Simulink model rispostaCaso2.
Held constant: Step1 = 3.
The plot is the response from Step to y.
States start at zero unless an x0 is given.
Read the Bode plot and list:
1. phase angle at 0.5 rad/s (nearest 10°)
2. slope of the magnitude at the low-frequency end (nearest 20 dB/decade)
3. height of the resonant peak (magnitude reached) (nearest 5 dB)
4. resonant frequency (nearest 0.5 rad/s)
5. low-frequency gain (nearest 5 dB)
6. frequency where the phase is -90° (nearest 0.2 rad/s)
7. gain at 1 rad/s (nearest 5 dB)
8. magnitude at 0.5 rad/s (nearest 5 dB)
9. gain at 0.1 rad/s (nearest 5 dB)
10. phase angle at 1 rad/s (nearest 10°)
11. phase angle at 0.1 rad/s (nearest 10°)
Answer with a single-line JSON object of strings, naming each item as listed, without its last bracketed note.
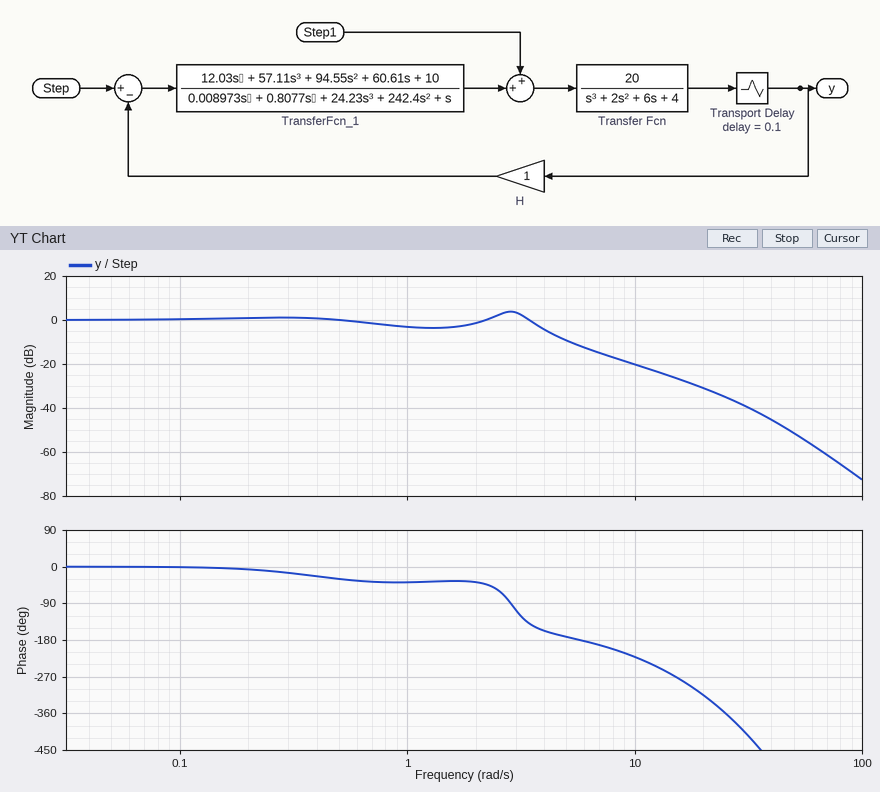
{"phase angle at 0.5 rad/s": "-30°", "slope of the magnitude at the low-frequency end": "0 dB/decade", "height of the resonant peak (magnitude reached)": "5 dB", "resonant frequency": "3.0 rad/s", "low-frequency gain": "0 dB", "frequency where the phase is -90°": "2.8 rad/s", "gain at 1 rad/s": "-5 dB", "magnitude at 0.5 rad/s": "0 dB", "gain at 0.1 rad/s": "0 dB", "phase angle at 1 rad/s": "-40°", "phase angle at 0.1 rad/s": "0°"}
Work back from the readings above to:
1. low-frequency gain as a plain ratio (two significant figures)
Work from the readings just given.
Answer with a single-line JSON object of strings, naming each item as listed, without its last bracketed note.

{"low-frequency gain as a plain ratio": "1.0"}
